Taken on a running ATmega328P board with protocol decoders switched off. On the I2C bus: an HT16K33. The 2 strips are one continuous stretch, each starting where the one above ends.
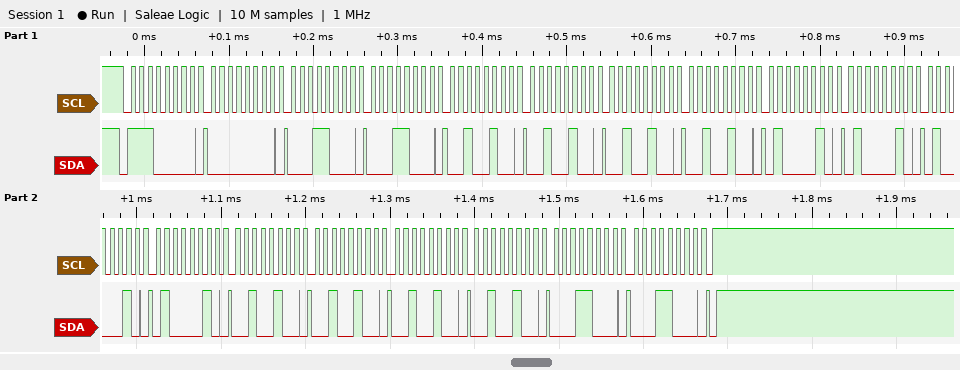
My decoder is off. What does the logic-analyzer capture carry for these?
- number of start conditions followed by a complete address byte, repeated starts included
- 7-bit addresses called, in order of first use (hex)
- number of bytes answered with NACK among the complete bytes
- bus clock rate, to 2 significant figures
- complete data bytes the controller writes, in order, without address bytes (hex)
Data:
1
0x70
0
100 kHz
00 18 18 24 24 24 24 42 42 42 42 24 24 24 24 18 18
